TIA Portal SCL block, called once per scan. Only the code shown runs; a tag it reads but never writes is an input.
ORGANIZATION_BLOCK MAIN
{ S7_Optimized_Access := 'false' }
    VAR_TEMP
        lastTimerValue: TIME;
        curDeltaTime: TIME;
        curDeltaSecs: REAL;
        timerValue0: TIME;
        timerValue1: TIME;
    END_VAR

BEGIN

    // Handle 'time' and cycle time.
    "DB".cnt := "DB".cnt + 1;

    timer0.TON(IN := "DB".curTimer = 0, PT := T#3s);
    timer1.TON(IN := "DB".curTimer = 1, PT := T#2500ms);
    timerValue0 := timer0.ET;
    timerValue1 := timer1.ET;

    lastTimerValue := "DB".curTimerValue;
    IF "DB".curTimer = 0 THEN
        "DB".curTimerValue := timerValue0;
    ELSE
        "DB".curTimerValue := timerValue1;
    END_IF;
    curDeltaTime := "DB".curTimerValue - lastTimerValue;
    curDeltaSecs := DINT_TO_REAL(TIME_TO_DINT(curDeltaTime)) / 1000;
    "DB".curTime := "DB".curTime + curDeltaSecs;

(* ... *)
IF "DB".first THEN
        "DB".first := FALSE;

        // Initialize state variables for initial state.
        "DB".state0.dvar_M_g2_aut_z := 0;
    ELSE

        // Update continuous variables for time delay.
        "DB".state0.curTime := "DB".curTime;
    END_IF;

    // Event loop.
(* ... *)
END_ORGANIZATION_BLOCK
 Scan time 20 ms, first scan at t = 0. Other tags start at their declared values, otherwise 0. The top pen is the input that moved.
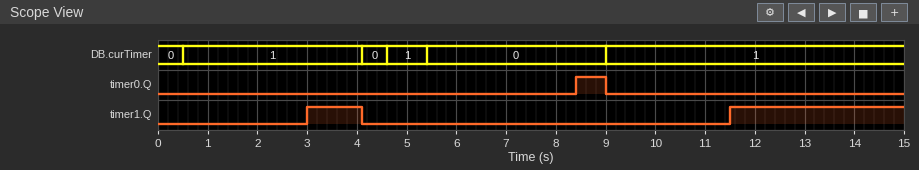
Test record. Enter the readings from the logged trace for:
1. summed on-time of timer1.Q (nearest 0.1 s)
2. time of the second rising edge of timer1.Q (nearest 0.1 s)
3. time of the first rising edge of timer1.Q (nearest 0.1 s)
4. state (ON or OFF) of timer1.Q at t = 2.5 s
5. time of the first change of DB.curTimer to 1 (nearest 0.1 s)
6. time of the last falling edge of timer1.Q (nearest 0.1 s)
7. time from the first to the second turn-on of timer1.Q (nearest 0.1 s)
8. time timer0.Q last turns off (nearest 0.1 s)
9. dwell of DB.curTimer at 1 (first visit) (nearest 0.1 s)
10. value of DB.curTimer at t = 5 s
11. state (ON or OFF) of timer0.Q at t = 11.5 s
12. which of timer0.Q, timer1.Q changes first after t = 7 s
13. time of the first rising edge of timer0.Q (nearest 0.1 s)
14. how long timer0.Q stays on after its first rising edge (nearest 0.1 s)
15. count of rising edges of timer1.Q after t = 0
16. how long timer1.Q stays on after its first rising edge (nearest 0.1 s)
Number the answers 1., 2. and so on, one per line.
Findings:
1. 4.6 s
2. 11.5 s
3. 3.0 s
4. OFF
5. 0.5 s
6. 4.1 s
7. 8.5 s
8. 9.0 s
9. 3.6 s
10. 1
11. OFF
12. timer0.Q
13. 8.4 s
14. 0.6 s
15. 2
16. 1.1 s
